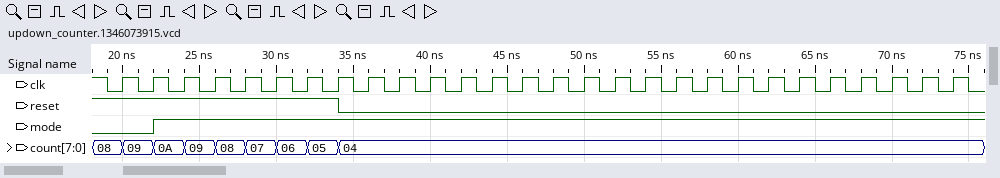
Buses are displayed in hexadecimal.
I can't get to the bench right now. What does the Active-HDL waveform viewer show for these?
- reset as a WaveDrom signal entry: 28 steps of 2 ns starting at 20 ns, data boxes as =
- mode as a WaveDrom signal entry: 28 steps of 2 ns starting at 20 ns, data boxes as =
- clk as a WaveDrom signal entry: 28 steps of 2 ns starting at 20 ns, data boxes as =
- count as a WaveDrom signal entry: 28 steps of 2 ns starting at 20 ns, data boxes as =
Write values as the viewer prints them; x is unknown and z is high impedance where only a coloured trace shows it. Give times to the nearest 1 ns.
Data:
{name: 'reset', wave: '1......0....................'}
{name: 'mode', wave: '01..........................'}
{name: 'clk', wave: 'p...........................'}
{name: 'count', wave: '========....................', data: '09 0A 09 08 07 06 05 04'}
